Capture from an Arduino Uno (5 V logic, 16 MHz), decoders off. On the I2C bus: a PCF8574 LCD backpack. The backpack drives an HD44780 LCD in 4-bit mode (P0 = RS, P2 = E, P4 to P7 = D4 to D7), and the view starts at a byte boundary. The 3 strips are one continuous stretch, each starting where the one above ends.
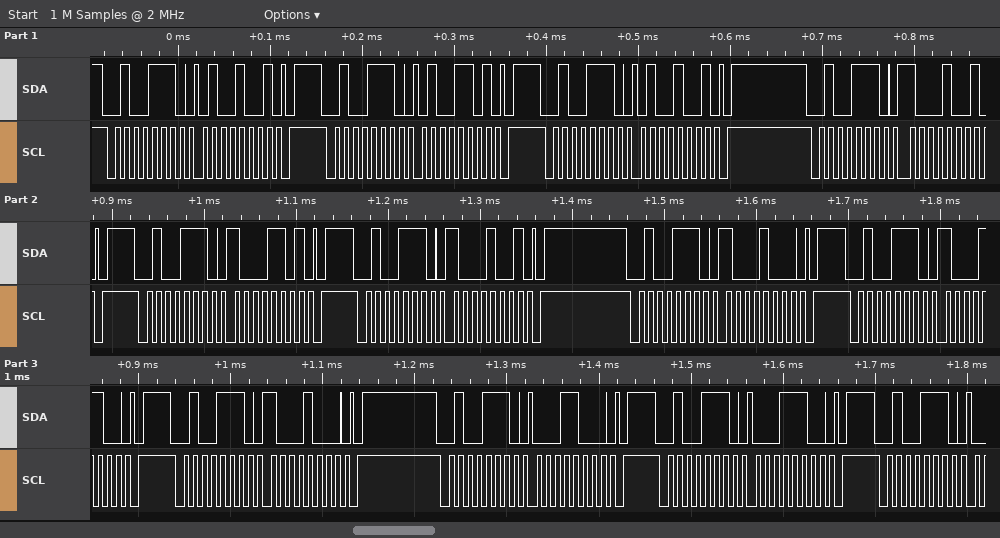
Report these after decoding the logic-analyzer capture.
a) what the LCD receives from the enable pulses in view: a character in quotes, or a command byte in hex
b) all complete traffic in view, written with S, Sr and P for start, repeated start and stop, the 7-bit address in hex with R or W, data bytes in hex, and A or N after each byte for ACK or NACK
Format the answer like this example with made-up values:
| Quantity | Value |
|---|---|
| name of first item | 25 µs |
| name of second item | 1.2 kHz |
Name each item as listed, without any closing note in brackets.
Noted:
| Quantity | Value |
|---|---|
| what the LCD receives from the enable pulses in view: a character in quotes, or a command byte in hex | 'H' |
| all complete traffic in view, written with S, Sr and P for start, repeated start and stop, the 7-bit address in hex with R or W, data bytes in hex, and A or N after each byte for ACK or NACK | S 27W A 49 A P S 27W A 4D A P S 27W A 49 A P S 27W A 89 A P S 27W A 8D A P S 27W A 89 A P S 27W A 88 A P S 27W A 8C A P S 27W A 88 A P S 27W A 18 A P S 27W A 1C A P S 27W A |
